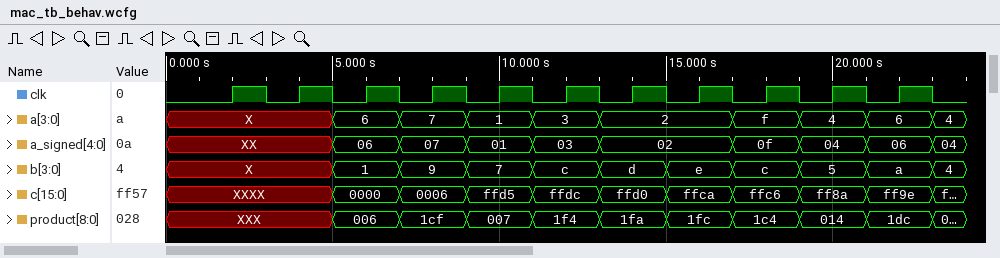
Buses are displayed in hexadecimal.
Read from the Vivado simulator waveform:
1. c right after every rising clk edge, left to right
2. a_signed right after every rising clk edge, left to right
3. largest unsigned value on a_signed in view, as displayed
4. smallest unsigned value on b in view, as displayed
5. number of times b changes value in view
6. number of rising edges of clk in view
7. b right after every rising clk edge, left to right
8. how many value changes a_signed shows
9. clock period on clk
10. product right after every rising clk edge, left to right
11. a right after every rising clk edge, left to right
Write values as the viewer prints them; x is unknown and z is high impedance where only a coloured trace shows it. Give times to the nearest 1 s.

XXXX, XXXX, 0000, 0006, ffd5, ffdc, ffd0, ffca, ffc6, ff8a, ff9e
XX, XX, 06, 07, 01, 03, 02, 02, 0f, 04, 06
0f
1
10
11
X, X, 1, 9, 7, c, d, e, c, 5, a
9
2 s
XXX, XXX, 006, 1cf, 007, 1f4, 1fa, 1fc, 1c4, 014, 1dc
X, X, 6, 7, 1, 3, 2, 2, f, 4, 6
